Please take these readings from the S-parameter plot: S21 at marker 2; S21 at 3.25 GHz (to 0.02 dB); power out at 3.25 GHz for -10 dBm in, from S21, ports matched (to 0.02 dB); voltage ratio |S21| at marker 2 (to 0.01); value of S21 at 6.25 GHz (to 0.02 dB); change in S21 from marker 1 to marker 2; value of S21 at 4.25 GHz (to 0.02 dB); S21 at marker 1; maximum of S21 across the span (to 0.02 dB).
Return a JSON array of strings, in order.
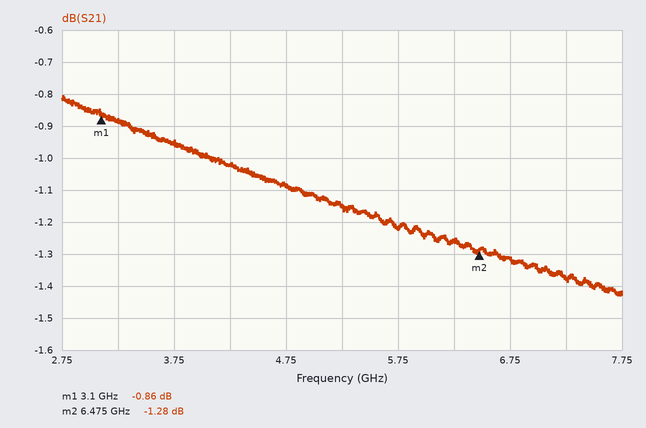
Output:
["-1.28 dB", "-0.88 dB", "-10.88 dBm", "0.86", "-1.26 dB", "-0.42 dB", "-1.02 dB", "-0.86 dB", "-0.80 dB"]
